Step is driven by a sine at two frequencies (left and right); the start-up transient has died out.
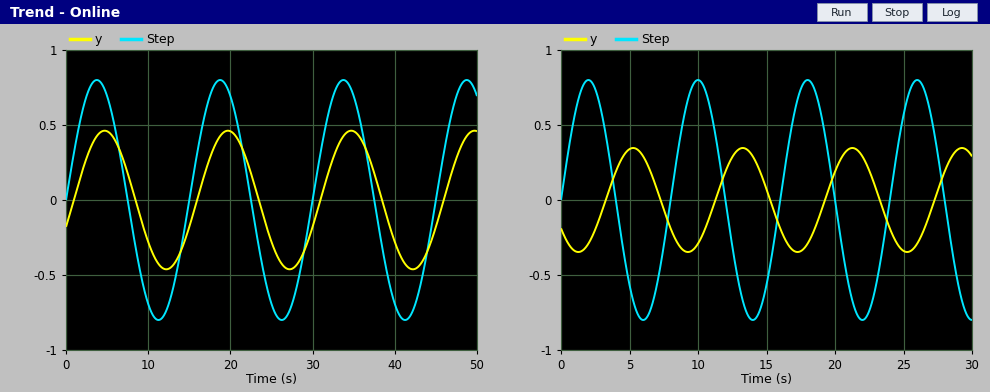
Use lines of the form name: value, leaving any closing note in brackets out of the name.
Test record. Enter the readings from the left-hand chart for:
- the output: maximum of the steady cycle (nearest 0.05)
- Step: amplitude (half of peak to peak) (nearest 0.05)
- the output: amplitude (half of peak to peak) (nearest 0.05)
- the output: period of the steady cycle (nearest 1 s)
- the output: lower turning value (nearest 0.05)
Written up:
the output: maximum of the steady cycle: 0.45
Step: amplitude (half of peak to peak): 0.80
the output: amplitude (half of peak to peak): 0.45
the output: period of the steady cycle: 15 s
the output: lower turning value: -0.45
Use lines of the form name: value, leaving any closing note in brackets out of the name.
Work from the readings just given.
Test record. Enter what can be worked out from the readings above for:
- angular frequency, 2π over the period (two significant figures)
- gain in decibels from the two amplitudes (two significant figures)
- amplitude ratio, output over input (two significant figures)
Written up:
angular frequency, 2π over the period: 0.42 rad/s
gain in decibels from the two amplitudes: -5.0 dB
amplitude ratio, output over input: 0.56
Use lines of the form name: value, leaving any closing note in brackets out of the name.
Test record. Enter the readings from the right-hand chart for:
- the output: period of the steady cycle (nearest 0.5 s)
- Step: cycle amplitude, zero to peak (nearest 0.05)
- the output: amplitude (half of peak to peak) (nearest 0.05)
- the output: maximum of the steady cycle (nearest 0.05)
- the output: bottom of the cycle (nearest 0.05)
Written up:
the output: period of the steady cycle: 8.0 s
Step: cycle amplitude, zero to peak: 0.80
the output: amplitude (half of peak to peak): 0.35
the output: maximum of the steady cycle: 0.35
the output: bottom of the cycle: -0.35
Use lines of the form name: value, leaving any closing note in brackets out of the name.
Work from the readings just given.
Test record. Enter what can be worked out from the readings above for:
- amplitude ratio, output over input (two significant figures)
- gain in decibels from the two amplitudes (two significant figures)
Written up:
amplitude ratio, output over input: 0.44
gain in decibels from the two amplitudes: -7.2 dB
